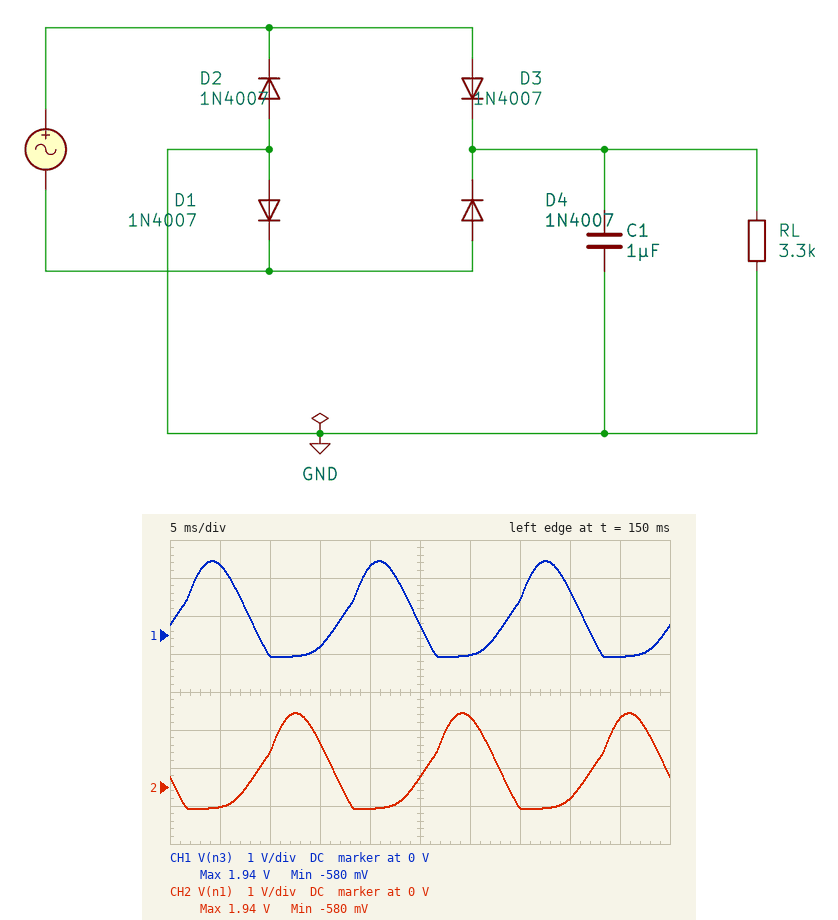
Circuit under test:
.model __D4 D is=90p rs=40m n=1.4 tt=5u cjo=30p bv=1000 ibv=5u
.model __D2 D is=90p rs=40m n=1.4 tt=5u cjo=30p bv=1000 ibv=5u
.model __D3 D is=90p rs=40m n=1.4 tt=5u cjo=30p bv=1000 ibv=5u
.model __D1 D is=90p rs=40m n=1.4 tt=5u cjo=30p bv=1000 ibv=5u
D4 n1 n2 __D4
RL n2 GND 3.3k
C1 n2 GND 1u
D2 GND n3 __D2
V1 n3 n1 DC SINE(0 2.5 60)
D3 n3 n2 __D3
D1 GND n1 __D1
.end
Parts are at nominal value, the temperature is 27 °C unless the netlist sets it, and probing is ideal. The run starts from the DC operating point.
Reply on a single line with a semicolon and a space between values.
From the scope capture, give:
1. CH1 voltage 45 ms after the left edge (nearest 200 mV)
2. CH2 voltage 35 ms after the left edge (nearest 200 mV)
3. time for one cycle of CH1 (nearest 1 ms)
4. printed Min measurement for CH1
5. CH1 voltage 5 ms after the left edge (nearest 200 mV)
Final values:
-600 mV; -600 mV; 17 ms; -580 mV; 1.8 V
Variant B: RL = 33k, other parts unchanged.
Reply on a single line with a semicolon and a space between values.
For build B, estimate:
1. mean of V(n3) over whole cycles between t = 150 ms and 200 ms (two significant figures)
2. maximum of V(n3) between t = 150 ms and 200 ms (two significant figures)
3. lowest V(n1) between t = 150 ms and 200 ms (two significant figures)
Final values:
680 mV; 2.0 V; -540 mV
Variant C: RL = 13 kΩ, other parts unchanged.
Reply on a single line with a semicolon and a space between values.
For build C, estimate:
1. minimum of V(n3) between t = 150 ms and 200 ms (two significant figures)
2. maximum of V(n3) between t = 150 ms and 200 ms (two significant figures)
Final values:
-560 mV; 2.0 V
